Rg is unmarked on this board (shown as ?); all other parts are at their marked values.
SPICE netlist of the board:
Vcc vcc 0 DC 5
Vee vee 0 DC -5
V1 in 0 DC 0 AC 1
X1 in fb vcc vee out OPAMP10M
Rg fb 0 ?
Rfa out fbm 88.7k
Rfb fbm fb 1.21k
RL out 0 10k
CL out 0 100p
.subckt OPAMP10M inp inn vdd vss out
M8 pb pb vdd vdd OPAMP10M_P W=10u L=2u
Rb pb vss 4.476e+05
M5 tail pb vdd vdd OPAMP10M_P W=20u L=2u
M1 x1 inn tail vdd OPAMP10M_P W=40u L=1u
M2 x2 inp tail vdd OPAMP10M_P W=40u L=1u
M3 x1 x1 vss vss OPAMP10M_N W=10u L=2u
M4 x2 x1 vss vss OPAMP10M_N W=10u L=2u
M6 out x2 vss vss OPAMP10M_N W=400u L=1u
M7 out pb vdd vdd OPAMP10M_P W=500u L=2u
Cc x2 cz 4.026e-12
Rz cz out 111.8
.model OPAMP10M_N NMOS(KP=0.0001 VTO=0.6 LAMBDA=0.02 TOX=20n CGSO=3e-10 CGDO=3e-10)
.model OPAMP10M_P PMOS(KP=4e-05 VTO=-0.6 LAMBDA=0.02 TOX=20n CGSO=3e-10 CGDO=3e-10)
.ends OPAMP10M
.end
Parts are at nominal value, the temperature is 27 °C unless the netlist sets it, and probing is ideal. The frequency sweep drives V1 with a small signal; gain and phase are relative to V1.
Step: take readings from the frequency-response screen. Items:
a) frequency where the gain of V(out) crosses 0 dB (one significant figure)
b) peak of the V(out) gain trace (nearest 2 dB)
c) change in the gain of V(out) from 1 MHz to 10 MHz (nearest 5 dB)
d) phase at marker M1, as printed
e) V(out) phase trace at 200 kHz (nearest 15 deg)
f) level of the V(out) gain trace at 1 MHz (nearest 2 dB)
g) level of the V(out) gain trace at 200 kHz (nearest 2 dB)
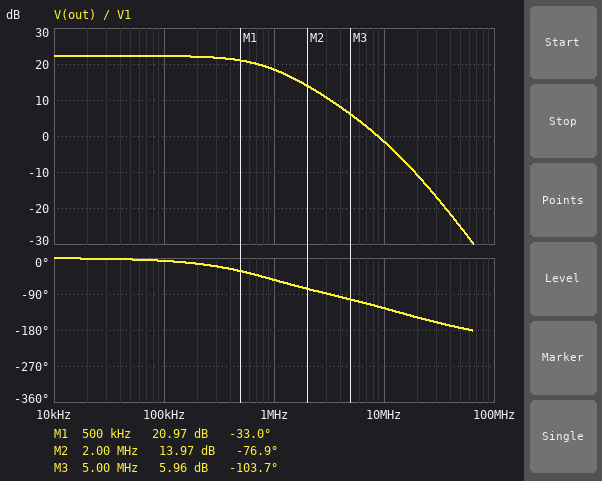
9 MHz
22 dB
-20 dB
-33.0 deg
-15 deg
18 dB
22 dB
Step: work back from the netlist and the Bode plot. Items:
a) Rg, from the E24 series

7.5 kΩ
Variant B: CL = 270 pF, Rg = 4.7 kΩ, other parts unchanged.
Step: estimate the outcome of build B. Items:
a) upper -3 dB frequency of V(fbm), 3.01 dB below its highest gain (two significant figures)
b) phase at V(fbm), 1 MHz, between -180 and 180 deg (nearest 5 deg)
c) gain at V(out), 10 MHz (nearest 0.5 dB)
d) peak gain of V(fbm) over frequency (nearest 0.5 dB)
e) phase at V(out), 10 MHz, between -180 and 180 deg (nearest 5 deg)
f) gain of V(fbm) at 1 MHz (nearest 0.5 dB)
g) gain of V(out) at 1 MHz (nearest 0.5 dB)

570 kHz
-75 deg
-6.5 dB
2.0 dB
-155 deg
-4.5 dB
20.0 dB
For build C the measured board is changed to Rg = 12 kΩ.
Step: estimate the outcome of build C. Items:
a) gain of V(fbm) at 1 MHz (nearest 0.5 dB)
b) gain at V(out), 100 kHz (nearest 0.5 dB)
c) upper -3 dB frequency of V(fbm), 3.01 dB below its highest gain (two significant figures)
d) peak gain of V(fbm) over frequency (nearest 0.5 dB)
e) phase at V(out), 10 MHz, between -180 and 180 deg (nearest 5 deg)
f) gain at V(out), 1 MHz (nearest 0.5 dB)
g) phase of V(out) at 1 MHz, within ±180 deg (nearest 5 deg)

-1.0 dB
18.5 dB
1.3 MHz
1.0 dB
-125 deg
16.5 dB
-40 deg
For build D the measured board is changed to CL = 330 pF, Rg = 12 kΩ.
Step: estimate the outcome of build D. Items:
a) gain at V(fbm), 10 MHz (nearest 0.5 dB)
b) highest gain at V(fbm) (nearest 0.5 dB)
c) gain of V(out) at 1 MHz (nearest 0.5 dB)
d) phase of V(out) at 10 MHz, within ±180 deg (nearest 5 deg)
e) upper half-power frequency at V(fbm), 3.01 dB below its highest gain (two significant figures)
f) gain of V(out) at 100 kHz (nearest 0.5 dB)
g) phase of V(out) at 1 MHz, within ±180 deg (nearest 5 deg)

-26.0 dB
1.0 dB
17.5 dB
-160 deg
1.6 MHz
18.5 dB
-45 deg
